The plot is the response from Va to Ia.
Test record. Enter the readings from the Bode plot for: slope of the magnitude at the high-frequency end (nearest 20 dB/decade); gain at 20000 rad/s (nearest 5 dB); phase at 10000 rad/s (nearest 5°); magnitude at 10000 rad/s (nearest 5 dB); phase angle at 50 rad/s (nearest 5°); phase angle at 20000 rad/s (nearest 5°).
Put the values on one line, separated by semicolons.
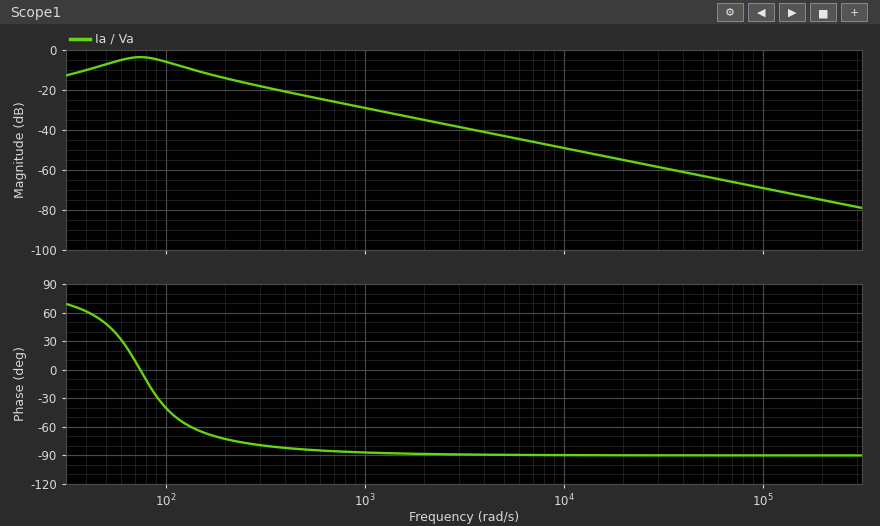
-20 dB/decade; -55 dB; -90°; -50 dB; 50°; -90°
